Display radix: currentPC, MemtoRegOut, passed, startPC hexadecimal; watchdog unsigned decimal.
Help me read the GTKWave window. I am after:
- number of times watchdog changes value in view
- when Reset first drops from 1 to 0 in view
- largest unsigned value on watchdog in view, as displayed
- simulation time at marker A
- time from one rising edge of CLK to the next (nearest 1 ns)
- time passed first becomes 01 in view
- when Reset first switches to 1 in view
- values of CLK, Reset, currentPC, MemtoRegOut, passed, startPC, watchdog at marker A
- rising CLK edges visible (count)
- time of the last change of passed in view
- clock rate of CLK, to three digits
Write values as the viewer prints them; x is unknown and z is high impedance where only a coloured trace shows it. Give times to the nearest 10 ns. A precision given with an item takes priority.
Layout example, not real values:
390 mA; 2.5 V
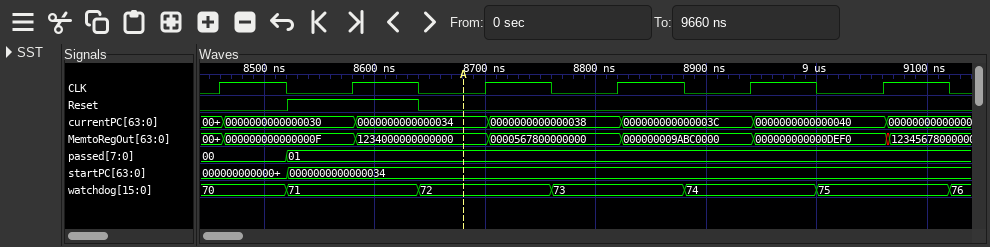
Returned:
6; 8640 ns; 76; 8680 ns; 120 ns; 8520 ns; 8520 ns; CLK=0, Reset=0, currentPC=0000000000000034, MemtoRegOut=1234000000000000, passed=01, startPC=0000000000000034, watchdog=72; 6; 8520 ns; 8.33 MHz
